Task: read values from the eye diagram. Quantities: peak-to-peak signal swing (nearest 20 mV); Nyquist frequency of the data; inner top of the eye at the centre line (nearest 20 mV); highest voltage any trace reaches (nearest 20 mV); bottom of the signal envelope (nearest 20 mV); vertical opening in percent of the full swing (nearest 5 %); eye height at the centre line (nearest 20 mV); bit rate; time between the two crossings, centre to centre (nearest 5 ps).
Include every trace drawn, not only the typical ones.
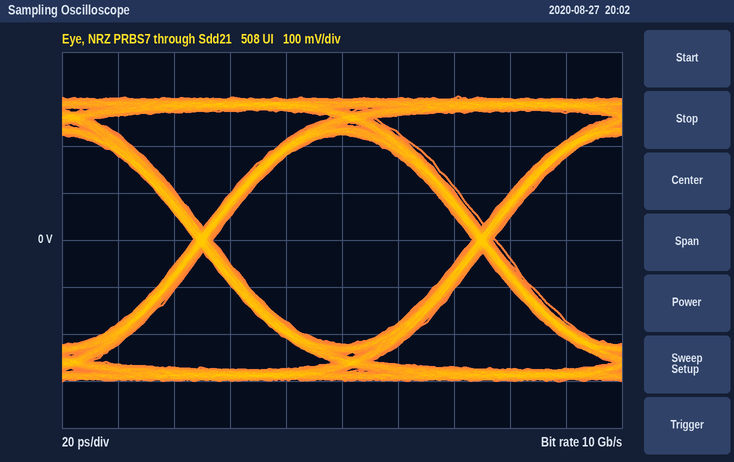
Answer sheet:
600 mV
5 GHz
220 mV
300 mV
-300 mV
75 %
440 mV
10 Gb/s
100 ps
